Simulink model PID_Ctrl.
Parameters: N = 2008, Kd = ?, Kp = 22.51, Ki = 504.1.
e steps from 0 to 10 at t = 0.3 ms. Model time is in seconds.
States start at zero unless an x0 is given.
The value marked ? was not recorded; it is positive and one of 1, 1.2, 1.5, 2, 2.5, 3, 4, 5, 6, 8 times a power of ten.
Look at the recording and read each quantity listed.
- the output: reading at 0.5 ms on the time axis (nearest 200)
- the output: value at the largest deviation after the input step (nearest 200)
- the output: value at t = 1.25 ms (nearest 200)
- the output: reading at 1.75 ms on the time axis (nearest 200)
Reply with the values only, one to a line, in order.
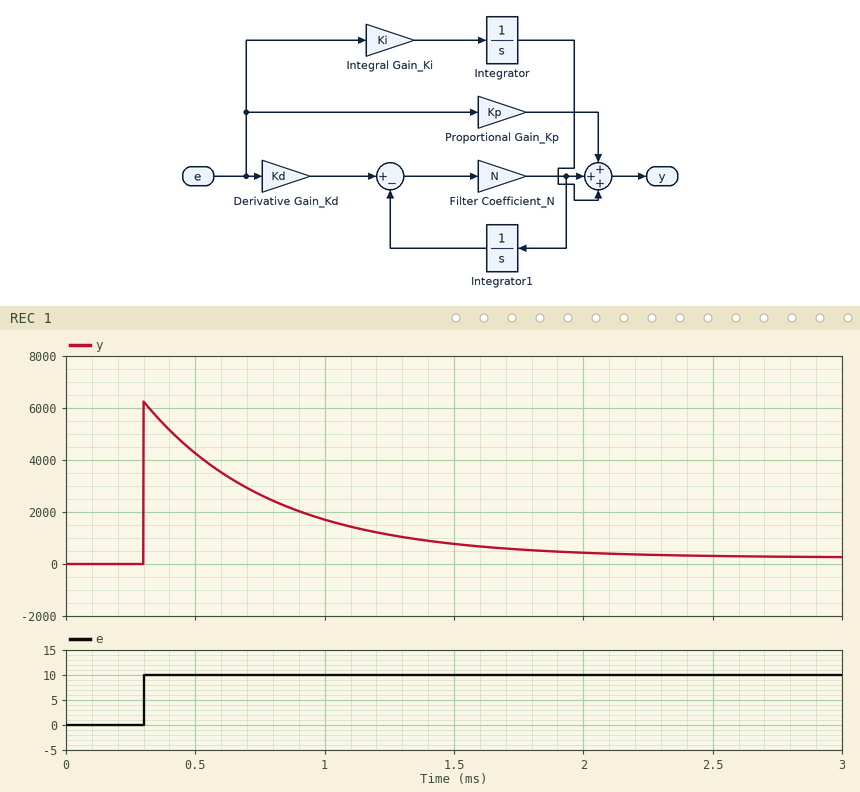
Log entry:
4200
6200
1200
600
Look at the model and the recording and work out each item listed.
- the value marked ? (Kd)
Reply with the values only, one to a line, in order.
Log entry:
0.3
